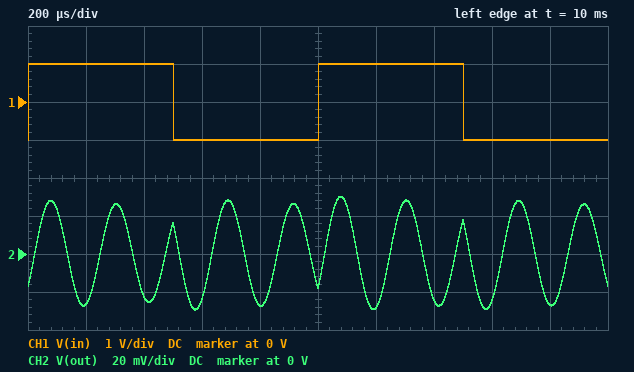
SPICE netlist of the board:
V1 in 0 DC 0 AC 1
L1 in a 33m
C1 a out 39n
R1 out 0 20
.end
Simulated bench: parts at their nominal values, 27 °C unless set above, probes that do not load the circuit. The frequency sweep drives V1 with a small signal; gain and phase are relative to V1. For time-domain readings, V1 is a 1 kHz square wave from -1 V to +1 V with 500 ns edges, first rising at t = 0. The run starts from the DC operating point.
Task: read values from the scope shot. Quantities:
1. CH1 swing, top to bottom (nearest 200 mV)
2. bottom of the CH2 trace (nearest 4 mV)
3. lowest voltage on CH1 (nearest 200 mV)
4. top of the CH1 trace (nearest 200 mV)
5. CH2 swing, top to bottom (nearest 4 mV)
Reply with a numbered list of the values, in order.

1. 2.0 V
2. -28 mV
3. -1.0 V
4. 1.0 V
5. 60 mV
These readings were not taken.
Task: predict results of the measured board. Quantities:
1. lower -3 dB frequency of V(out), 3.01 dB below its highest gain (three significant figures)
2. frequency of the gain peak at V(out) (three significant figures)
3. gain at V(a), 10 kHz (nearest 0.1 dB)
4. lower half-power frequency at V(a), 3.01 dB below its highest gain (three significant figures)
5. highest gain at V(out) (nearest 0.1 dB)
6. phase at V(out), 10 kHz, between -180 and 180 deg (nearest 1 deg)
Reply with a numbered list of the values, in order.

1. 4.39 kHz
2. 4.44 kHz
3. -12.2 dB
4. 4.39 kHz
5. 0 dB
6. -89 deg
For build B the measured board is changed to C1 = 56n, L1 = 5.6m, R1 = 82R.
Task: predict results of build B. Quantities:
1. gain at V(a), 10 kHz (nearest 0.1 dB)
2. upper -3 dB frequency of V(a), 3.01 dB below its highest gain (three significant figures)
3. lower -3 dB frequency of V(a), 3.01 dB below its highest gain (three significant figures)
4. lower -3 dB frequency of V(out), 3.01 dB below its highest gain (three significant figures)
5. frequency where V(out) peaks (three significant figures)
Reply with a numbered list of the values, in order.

1. 8.9 dB
2. 9.96 kHz
3. 7.59 kHz
4. 7.90 kHz
5. 8.99 kHz
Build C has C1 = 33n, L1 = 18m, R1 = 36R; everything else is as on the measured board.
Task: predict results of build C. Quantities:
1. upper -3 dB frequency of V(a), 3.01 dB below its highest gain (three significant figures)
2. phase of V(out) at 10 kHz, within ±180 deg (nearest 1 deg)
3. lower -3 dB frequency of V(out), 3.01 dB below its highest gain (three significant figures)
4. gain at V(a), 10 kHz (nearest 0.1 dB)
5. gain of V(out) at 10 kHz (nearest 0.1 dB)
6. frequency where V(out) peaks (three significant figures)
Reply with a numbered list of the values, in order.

1. 6.68 kHz
2. -87 deg
3. 6.37 kHz
4. -2.6 dB
5. -25.1 dB
6. 6.53 kHz
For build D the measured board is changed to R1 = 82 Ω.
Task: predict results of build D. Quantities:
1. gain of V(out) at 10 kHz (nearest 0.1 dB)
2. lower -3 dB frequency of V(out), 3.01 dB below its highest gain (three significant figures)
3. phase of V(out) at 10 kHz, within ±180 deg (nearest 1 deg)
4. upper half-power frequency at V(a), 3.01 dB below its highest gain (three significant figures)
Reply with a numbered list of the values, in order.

1. -26.2 dB
2. 4.24 kHz
3. -87 deg
4. 4.62 kHz
